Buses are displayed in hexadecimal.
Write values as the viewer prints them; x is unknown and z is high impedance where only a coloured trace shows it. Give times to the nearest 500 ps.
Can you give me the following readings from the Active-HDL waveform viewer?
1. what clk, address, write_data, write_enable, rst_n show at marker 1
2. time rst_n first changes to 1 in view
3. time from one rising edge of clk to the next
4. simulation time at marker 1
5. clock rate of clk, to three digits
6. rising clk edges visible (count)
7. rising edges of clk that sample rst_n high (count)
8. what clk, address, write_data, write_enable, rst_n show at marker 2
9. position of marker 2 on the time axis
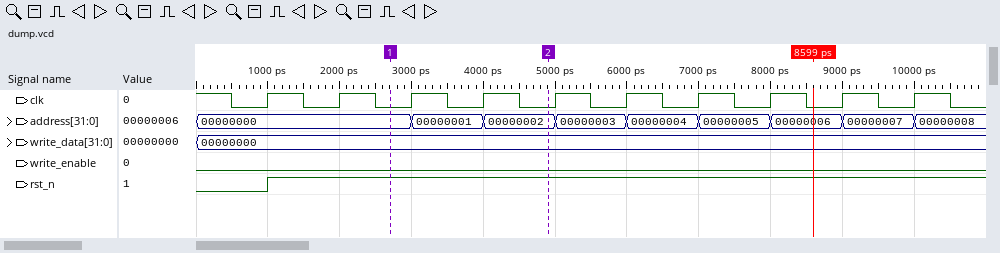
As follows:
clk=0, address=00000000, write_data=00000000, write_enable=0, rst_n=1
1000 ps
1000 ps
2500 ps
1.00 GHz
10
9
clk=0, address=00000002, write_data=00000000, write_enable=0, rst_n=1
5000 ps
